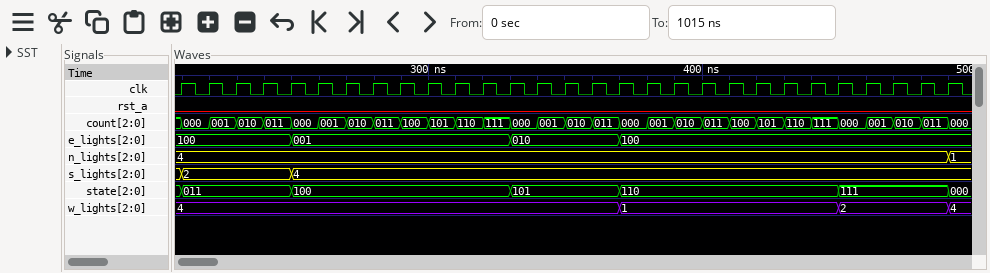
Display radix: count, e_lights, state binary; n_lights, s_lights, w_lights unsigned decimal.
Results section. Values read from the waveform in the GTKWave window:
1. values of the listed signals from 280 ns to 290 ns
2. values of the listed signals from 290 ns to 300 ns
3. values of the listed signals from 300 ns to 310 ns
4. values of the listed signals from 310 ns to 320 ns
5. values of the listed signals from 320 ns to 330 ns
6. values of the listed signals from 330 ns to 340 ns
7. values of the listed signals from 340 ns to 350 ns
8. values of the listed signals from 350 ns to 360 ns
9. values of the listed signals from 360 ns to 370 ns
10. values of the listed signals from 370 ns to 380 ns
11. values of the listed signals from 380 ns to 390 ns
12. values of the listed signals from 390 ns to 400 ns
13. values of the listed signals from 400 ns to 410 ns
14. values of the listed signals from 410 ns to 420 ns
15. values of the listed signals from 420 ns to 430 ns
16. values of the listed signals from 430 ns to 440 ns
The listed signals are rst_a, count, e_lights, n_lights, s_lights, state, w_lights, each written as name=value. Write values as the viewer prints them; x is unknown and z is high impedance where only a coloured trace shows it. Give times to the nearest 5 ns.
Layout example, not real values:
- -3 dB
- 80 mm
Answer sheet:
- rst_a=0, count=011, e_lights=001, n_lights=4, s_lights=4, state=100, w_lights=4
- rst_a=0, count=100, e_lights=001, n_lights=4, s_lights=4, state=100, w_lights=4
- rst_a=0, count=101, e_lights=001, n_lights=4, s_lights=4, state=100, w_lights=4
- rst_a=0, count=110, e_lights=001, n_lights=4, s_lights=4, state=100, w_lights=4
- rst_a=0, count=111, e_lights=001, n_lights=4, s_lights=4, state=100, w_lights=4
- rst_a=0, count=000, e_lights=010, n_lights=4, s_lights=4, state=101, w_lights=4
- rst_a=0, count=001, e_lights=010, n_lights=4, s_lights=4, state=101, w_lights=4
- rst_a=0, count=010, e_lights=010, n_lights=4, s_lights=4, state=101, w_lights=4
- rst_a=0, count=011, e_lights=010, n_lights=4, s_lights=4, state=101, w_lights=4
- rst_a=0, count=000, e_lights=100, n_lights=4, s_lights=4, state=110, w_lights=1
- rst_a=0, count=001, e_lights=100, n_lights=4, s_lights=4, state=110, w_lights=1
- rst_a=0, count=010, e_lights=100, n_lights=4, s_lights=4, state=110, w_lights=1
- rst_a=0, count=011, e_lights=100, n_lights=4, s_lights=4, state=110, w_lights=1
- rst_a=0, count=100, e_lights=100, n_lights=4, s_lights=4, state=110, w_lights=1
- rst_a=0, count=101, e_lights=100, n_lights=4, s_lights=4, state=110, w_lights=1
- rst_a=0, count=110, e_lights=100, n_lights=4, s_lights=4, state=110, w_lights=1
